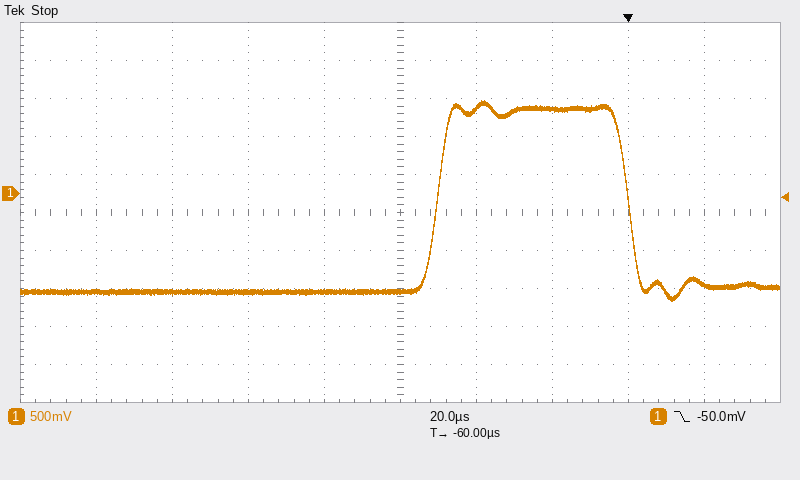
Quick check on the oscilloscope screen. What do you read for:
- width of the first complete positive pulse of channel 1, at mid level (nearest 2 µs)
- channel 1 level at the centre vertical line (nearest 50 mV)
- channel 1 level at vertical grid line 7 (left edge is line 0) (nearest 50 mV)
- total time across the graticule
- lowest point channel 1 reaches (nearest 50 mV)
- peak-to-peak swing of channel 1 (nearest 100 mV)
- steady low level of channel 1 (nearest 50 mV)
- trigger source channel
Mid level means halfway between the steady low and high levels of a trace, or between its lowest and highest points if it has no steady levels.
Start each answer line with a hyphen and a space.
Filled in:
- 50 µs
- -1.30 V
- 1.10 V
- 200 µs
- -1.40 V
- 2.60 V
- -1.30 V
- channel 1
